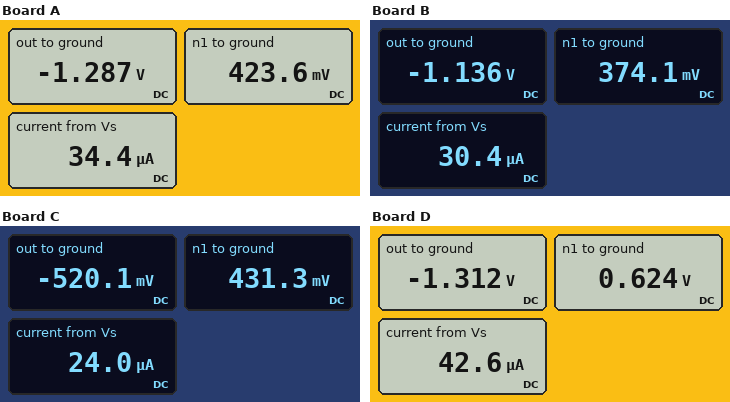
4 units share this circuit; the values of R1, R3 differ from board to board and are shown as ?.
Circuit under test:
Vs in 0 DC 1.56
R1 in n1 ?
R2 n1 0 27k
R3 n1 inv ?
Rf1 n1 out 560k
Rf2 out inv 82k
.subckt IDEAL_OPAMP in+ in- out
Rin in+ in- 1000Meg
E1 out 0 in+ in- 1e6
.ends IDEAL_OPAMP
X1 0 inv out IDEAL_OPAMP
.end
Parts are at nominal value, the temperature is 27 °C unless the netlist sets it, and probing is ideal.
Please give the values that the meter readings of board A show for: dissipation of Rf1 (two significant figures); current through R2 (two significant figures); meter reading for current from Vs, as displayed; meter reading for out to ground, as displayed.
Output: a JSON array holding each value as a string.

["5.2 µW", "16 µA", "34.4 µA", "-1.287 V"]
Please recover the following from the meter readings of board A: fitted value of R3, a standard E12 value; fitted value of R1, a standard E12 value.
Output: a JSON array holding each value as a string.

["27 kΩ", "33 kΩ"]
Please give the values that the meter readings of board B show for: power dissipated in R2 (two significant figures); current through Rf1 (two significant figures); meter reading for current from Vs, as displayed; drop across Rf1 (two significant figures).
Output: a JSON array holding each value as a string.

["5.2 µW", "2.7 µA", "30.4 µA", "1.5 V"]
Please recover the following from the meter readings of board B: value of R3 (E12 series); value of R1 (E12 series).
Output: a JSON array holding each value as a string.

["27 kΩ", "39 kΩ"]
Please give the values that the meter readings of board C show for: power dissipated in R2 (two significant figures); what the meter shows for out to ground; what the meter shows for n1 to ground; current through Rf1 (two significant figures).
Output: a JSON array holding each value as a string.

["6.9 µW", "-520.1 mV", "431.3 mV", "1.7 µA"]
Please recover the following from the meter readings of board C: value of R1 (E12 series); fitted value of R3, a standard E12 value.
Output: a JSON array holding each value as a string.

["47 kΩ", "68 kΩ"]
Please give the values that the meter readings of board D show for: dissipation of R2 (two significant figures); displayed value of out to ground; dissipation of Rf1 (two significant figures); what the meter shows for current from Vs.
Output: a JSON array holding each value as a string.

["14 µW", "-1.312 V", "6.7 µW", "42.6 µA"]
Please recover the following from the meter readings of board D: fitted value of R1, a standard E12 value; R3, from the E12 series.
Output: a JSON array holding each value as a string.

["22 kΩ", "39 kΩ"]
